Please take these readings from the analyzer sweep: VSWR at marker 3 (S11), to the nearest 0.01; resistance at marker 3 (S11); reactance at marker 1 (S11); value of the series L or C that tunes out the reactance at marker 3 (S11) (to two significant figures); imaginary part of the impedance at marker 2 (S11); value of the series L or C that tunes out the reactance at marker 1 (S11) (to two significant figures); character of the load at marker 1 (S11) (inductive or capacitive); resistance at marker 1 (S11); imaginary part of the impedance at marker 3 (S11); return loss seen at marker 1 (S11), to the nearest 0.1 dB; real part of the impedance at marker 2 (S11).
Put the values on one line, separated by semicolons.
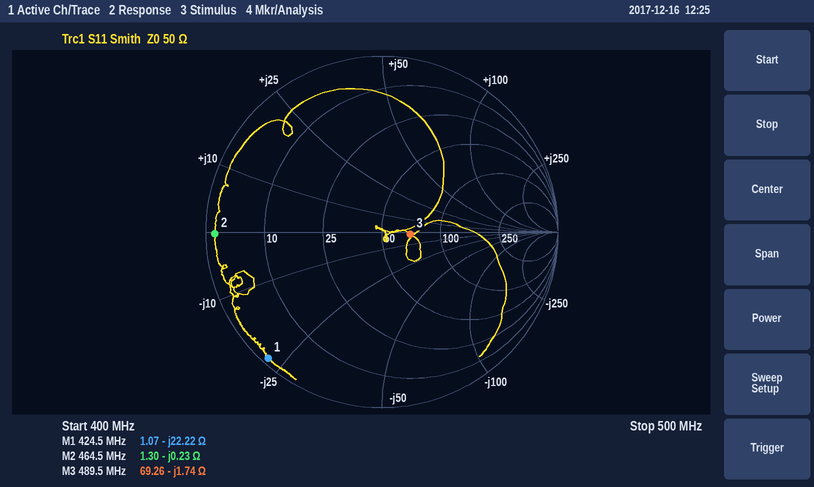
1.39; 69.26 Ω; -22.22 Ω; 570 pH; -0.23 Ω; 8.3 nH; capacitive; 1.07 Ω; -1.74 Ω; 0.3 dB; 1.30 Ω
